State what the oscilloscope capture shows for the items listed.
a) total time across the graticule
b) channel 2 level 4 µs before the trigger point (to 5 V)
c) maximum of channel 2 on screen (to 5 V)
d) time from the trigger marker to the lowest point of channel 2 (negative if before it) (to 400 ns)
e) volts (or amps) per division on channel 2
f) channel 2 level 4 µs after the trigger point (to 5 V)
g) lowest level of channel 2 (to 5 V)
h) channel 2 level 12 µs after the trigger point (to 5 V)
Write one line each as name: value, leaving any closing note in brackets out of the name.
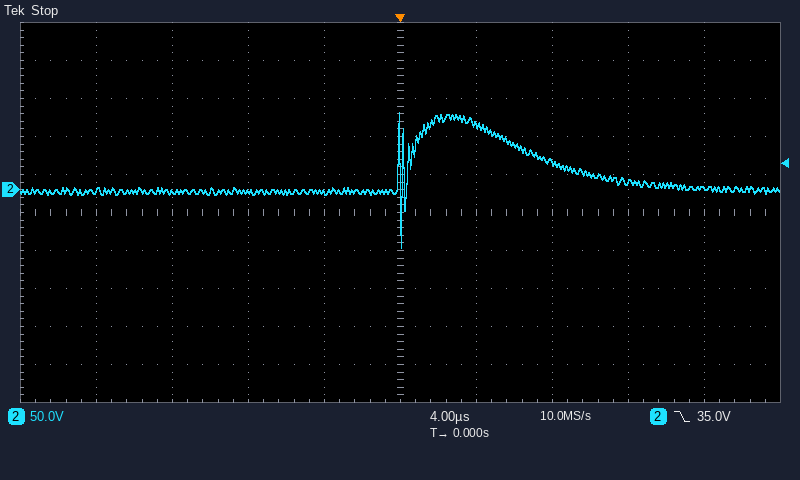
total time across the graticule: 40 µs
channel 2 level 4 µs before the trigger point: -5 V
maximum of channel 2 on screen: 100 V
time from the trigger marker to the lowest point of channel 2 (negative if before it): 0.0 µs
volts (or amps) per division on channel 2: 50 V
channel 2 level 4 µs after the trigger point: 85 V
lowest level of channel 2: -75 V
channel 2 level 12 µs after the trigger point: 10 V
